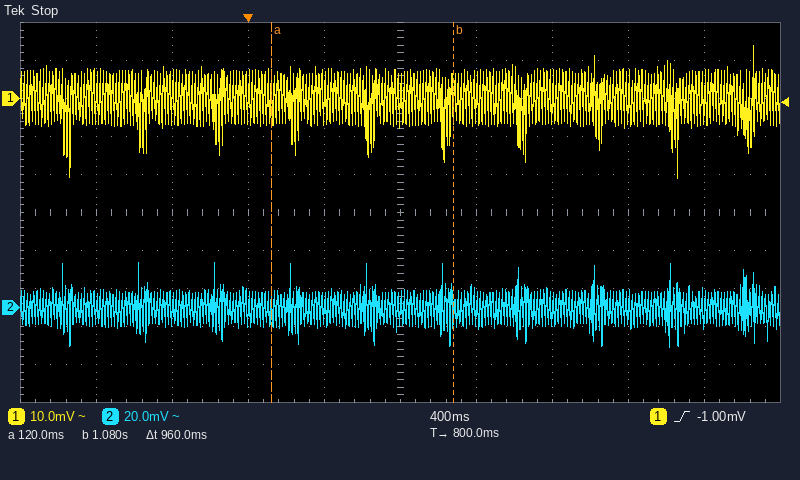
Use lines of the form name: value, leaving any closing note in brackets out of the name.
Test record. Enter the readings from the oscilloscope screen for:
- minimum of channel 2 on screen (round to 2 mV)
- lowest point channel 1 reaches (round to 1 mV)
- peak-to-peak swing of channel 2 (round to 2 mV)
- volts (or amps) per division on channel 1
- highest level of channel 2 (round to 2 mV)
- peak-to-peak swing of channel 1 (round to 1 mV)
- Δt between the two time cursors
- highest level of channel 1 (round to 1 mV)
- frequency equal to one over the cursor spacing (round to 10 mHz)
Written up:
minimum of channel 2 on screen: -20 mV
lowest point channel 1 reaches: -21 mV
peak-to-peak swing of channel 2: 44 mV
volts (or amps) per division on channel 1: 10 mV
highest level of channel 2: 24 mV
peak-to-peak swing of channel 1: 35 mV
Δt between the two time cursors: 960 ms
highest level of channel 1: 14 mV
frequency equal to one over the cursor spacing: 1.04 Hz
